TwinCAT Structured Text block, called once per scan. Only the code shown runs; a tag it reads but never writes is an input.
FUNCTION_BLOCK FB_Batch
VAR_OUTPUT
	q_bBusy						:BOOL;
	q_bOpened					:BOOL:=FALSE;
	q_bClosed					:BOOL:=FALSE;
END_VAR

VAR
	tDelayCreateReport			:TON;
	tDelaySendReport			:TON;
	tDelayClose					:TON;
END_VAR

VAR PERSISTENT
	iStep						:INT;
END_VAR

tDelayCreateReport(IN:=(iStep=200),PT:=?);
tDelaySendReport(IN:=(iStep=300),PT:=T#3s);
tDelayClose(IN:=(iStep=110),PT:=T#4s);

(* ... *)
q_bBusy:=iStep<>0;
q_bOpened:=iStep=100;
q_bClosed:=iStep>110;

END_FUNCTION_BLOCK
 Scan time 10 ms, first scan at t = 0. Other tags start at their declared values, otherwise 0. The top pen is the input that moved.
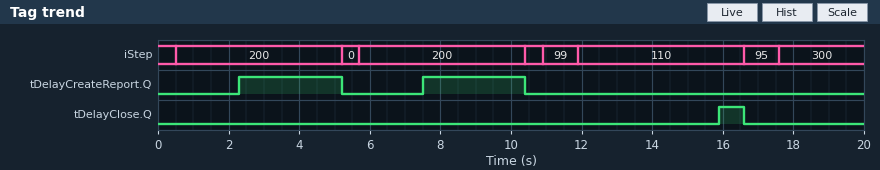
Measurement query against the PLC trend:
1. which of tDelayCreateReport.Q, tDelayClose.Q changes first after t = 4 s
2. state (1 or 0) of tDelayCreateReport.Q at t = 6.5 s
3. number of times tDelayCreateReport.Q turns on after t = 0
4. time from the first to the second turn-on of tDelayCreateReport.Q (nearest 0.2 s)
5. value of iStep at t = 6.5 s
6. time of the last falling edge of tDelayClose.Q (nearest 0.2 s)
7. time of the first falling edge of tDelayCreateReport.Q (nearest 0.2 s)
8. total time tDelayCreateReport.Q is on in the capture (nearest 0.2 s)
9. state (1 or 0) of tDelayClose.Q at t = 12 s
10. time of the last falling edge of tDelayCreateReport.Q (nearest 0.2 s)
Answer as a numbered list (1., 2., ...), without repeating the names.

1. tDelayCreateReport.Q
2. 0
3. 2
4. 5.2 s
5. 200
6. 16.6 s
7. 5.2 s
8. 5.8 s
9. 0
10. 10.4 s
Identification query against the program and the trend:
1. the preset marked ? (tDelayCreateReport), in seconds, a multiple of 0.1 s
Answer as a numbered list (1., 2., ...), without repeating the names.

1. 1.8 s
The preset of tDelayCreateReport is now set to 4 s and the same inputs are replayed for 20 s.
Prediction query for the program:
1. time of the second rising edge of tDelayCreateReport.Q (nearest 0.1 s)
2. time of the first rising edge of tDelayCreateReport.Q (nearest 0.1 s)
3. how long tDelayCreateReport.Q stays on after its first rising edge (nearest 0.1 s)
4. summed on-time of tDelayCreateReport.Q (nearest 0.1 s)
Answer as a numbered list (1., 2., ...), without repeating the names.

1. 9.7 s
2. 4.5 s
3. 0.7 s
4. 1.4 s
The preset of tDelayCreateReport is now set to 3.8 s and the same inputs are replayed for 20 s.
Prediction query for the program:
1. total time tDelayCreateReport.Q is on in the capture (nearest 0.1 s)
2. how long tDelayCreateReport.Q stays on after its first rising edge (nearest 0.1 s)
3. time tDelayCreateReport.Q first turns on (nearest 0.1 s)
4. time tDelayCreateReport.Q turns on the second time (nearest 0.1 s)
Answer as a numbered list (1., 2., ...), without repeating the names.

1. 1.8 s
2. 0.9 s
3. 4.3 s
4. 9.5 s
